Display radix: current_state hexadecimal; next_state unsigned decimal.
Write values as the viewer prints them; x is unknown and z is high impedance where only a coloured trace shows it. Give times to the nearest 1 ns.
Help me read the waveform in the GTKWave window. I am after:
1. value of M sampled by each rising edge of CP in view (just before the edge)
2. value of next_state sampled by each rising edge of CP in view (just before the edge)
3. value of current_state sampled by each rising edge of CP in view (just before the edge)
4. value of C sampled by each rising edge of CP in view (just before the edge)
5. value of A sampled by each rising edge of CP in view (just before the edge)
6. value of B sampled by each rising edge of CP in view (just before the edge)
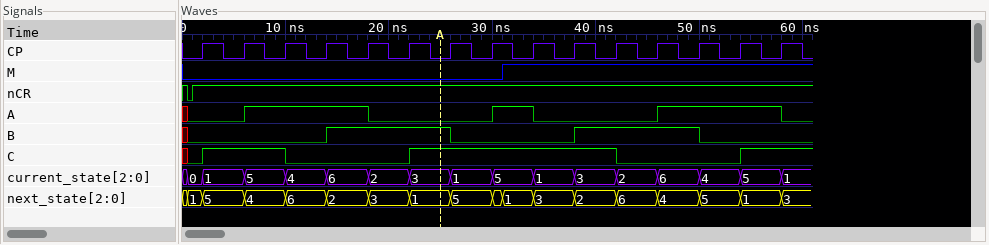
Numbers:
0 0 0 0 0 0 0 0 1 1 1 1 1 1 1
1, 5, 4, 6, 2, 3, 1, 5, 1, 3, 2, 6, 4, 5, 1
0, 1, 5, 4, 6, 2, 3, 1, 5, 1, 3, 2, 6, 4, 5
0 1 1 0 0 0 1 1 1 1 1 0 0 0 1
0 0 1 1 1 0 0 0 1 0 0 0 1 1 1
0 0 0 0 1 1 1 0 0 0 1 1 1 0 0
